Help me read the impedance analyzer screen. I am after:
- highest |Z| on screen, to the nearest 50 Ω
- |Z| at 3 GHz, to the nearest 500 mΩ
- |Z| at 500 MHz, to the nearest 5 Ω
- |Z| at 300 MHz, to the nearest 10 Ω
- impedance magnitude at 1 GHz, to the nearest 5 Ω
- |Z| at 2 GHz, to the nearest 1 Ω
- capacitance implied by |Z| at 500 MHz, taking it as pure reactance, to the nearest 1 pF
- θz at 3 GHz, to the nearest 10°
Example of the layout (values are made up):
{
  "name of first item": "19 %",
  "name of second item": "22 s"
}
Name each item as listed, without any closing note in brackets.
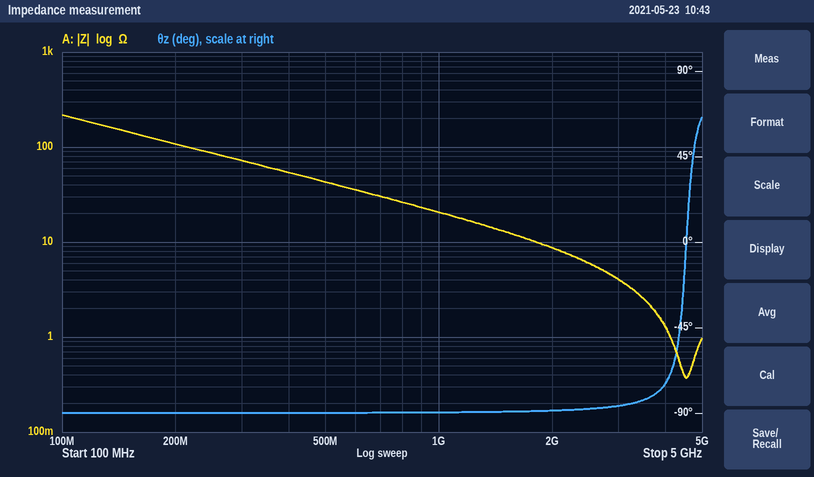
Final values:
{
  "highest |Z| on screen, to the nearest 50 Ω": "200 Ω",
  "|Z| at 3 GHz, to the nearest 500 mΩ": "4.0 Ω",
  "|Z| at 500 MHz, to the nearest 5 Ω": "45 Ω",
  "|Z| at 300 MHz, to the nearest 10 Ω": "70 Ω",
  "impedance magnitude at 1 GHz, to the nearest 5 Ω": "20 Ω",
  "|Z| at 2 GHz, to the nearest 1 Ω": "9 Ω",
  "capacitance implied by |Z| at 500 MHz, taking it as pure reactance, to the nearest 1 pF": "7 pF",
  "θz at 3 GHz, to the nearest 10°": "-90°"
}
